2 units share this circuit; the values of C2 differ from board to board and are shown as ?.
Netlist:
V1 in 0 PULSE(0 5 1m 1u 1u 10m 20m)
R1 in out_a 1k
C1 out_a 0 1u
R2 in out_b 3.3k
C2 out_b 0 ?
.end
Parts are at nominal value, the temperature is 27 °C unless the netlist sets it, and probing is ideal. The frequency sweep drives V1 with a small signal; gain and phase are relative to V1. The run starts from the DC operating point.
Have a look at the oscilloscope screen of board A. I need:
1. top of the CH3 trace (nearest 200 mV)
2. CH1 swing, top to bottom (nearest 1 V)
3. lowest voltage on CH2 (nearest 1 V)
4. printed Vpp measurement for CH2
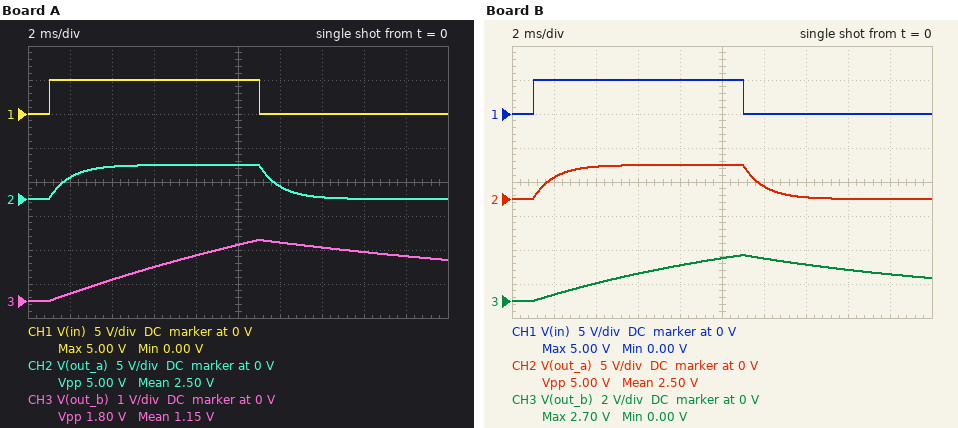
1.8 V
5 V
0 V
5.00 V
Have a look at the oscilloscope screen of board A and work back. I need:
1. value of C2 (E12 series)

6.8 µF
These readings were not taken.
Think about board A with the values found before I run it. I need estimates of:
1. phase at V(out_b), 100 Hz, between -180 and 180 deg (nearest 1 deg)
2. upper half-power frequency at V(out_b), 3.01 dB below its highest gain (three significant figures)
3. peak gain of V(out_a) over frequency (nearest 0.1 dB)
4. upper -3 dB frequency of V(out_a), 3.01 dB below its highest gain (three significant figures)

-86 deg
7.09 Hz
0 dB
159 Hz
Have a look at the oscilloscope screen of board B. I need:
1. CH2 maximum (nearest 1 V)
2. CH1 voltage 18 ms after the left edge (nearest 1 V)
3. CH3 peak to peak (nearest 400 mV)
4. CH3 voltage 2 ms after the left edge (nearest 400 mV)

5 V
0 V
2.8 V
400 mV
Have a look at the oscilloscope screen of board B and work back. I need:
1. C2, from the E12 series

3.9 µF
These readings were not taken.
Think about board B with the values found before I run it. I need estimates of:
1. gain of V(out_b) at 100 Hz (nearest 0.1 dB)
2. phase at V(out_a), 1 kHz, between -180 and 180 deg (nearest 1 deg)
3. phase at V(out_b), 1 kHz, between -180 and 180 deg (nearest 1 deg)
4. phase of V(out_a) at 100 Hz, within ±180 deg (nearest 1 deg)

-18.2 dB
-81 deg
-89 deg
-32 deg
